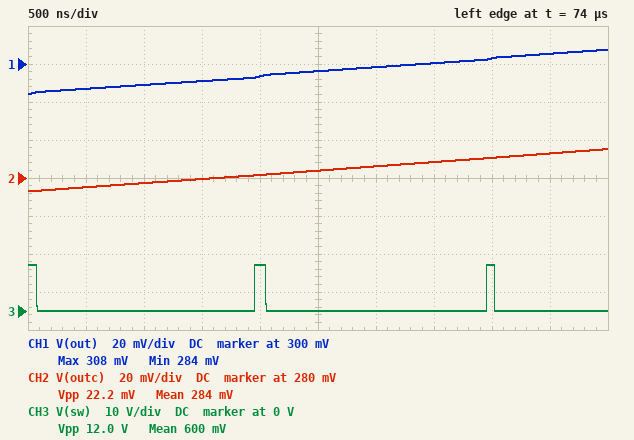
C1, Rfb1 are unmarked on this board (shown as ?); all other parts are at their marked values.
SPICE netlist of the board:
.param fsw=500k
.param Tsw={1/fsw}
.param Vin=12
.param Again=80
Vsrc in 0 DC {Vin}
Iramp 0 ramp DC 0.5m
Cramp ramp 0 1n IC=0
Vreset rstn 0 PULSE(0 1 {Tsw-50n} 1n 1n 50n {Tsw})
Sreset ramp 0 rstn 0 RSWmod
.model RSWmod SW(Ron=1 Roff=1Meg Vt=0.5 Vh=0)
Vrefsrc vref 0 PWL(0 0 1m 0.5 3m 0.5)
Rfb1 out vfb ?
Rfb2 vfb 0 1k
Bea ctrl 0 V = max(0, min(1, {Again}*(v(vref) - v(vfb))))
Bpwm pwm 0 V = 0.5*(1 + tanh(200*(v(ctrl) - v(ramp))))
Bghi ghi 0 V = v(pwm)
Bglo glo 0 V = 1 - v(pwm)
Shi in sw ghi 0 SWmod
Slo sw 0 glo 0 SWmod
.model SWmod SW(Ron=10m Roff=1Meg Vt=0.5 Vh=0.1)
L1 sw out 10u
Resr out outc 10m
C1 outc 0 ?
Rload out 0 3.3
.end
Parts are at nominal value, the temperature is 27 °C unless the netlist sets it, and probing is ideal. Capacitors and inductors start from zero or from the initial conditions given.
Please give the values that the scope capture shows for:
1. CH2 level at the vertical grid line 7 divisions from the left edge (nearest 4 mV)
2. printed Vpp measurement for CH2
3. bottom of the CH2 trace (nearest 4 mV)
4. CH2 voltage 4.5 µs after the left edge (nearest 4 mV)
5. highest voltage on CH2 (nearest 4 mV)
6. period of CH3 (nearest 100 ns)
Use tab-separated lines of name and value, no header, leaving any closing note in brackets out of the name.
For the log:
CH2 level at the vertical grid line 7 divisions from the left edge	288 mV
printed Vpp measurement for CH2	22.2 mV
bottom of the CH2 trace	272 mV
CH2 voltage 4.5 µs after the left edge	292 mV
highest voltage on CH2	296 mV
period of CH3	2.0 µs
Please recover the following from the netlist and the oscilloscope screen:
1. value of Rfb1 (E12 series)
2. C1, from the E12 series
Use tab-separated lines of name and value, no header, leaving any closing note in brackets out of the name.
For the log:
value of Rfb1	6.8 kΩ
C1, from the E12 series	270 µF
